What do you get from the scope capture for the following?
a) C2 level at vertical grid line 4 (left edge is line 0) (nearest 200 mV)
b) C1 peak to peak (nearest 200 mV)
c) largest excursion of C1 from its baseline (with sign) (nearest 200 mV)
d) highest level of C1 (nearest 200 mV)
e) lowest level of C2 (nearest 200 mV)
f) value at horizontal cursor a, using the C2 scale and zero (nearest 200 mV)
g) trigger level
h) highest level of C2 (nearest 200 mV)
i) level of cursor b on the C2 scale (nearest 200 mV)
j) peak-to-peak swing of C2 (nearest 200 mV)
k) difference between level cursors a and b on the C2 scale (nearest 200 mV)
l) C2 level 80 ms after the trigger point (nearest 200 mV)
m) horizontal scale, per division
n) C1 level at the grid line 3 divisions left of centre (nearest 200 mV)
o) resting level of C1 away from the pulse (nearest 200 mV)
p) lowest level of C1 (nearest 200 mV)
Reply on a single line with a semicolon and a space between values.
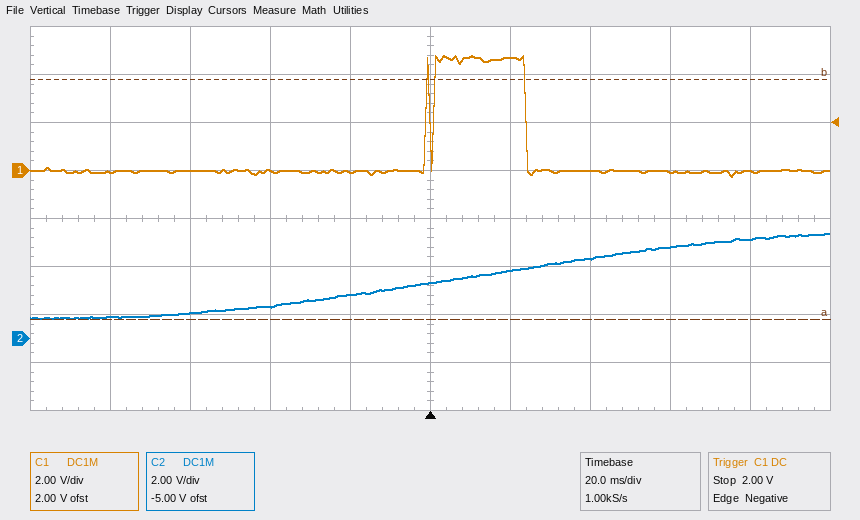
1.8 V; 5.0 V; +4.8 V; 4.8 V; 800 mV; 800 mV; 2.00 V; 4.4 V; 10.8 V; 3.6 V; 10.0 V; 4.2 V; 20 ms; 0.0 V; 0.0 V; -200 mV
